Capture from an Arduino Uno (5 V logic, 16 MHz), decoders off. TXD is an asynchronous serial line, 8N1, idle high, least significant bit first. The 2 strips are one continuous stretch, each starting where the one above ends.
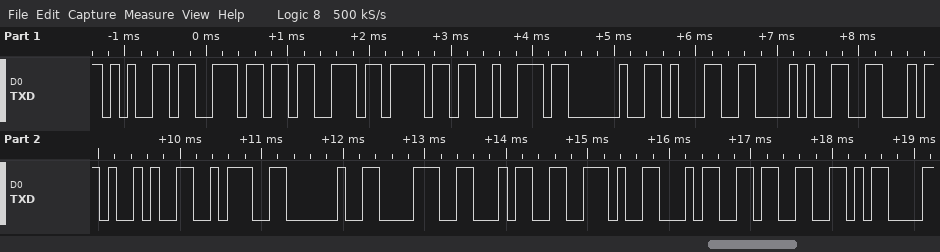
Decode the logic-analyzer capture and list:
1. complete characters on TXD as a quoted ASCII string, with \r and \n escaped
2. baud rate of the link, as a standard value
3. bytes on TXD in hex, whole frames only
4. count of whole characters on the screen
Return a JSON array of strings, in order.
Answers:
["\"ensor 1(F): 84.43\\r\"", "9600 baud", "65 6E 73 6F 72 20 31 28 46 29 3A 20 38 34 2E 34 33 0D", "18"]
